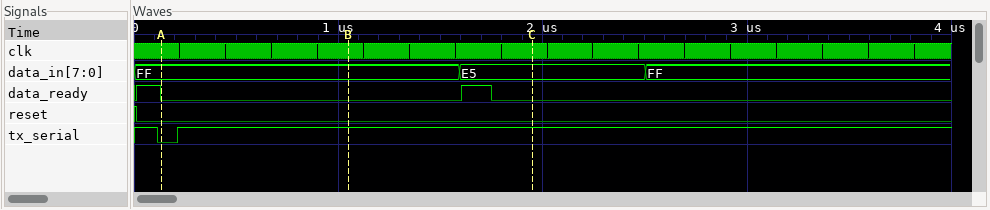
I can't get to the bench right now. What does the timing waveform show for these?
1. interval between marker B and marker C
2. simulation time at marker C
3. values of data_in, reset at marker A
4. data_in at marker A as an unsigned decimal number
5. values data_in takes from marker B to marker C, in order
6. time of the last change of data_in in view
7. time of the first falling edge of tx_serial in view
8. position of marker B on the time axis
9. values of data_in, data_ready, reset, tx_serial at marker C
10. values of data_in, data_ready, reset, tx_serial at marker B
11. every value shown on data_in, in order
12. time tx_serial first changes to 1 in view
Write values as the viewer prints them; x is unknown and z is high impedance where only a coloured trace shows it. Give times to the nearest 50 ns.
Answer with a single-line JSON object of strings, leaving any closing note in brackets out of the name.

{"interval between marker B and marker C": "900 ns", "simulation time at marker C": "1950 ns", "values of data_in, reset at marker A": "data_in=FF, reset=0", "data_in at marker A as an unsigned decimal number": "255", "values data_in takes from marker B to marker C, in order": "FF, E5", "time of the last change of data_in in view": "2500 ns", "time of the first falling edge of tx_serial in view": "100 ns", "position of marker B on the time axis": "1050 ns", "values of data_in, data_ready, reset, tx_serial at marker C": "data_in=E5, data_ready=0, reset=0, tx_serial=1", "values of data_in, data_ready, reset, tx_serial at marker B": "data_in=FF, data_ready=0, reset=0, tx_serial=1", "every value shown on data_in, in order": "FF, E5, FF", "time tx_serial first changes to 1 in view": "200 ns"}
